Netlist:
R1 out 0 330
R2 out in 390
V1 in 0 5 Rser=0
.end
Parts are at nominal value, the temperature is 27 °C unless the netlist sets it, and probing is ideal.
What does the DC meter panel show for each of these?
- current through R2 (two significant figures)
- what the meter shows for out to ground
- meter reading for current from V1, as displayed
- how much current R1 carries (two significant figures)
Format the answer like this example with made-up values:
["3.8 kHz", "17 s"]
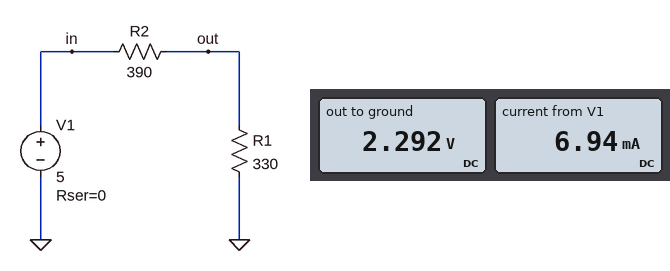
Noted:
["6.9 mA", "2.292 V", "6.94 mA", "6.9 mA"]
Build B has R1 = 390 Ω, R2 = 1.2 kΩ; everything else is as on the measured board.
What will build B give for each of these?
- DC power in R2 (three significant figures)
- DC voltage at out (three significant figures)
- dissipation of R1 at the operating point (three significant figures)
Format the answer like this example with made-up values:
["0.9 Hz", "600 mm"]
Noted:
["11.9 mW", "1.23 V", "3.86 mW"]
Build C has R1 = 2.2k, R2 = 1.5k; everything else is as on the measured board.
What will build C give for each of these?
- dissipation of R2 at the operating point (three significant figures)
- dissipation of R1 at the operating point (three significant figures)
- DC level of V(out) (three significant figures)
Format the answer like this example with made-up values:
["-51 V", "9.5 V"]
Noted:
["2.74 mW", "4.02 mW", "2.97 V"]
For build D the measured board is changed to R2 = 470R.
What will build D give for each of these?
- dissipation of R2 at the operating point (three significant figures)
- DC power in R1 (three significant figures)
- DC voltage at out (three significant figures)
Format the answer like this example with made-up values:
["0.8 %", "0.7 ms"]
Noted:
["18.4 mW", "12.9 mW", "2.06 V"]
